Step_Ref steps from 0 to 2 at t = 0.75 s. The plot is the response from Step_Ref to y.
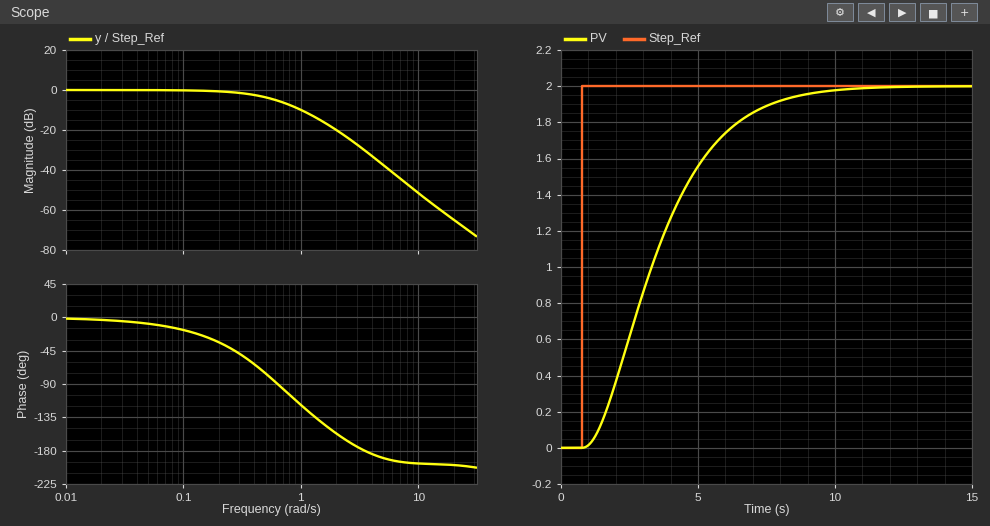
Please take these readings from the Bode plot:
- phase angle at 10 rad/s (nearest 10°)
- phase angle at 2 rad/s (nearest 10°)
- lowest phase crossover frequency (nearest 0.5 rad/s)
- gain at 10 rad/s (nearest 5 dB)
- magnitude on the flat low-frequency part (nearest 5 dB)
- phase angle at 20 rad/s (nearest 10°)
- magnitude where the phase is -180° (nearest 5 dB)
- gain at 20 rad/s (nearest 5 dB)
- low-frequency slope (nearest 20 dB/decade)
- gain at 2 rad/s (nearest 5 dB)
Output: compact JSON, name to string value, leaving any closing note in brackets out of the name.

{"phase angle at 10 rad/s": "-200°", "phase angle at 2 rad/s": "-160°", "lowest phase crossover frequency": "3.5 rad/s", "gain at 10 rad/s": "-50 dB", "magnitude on the flat low-frequency part": "0 dB", "phase angle at 20 rad/s": "-200°", "magnitude where the phase is -180°": "-30 dB", "gain at 20 rad/s": "-65 dB", "low-frequency slope": "0 dB/decade", "gain at 2 rad/s": "-20 dB"}
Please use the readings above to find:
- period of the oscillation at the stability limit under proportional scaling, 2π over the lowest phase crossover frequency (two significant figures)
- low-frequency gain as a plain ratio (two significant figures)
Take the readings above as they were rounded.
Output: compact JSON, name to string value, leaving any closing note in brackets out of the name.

{"period of the oscillation at the stability limit under proportional scaling, 2π over the lowest phase crossover frequency": "1.8 s", "low-frequency gain as a plain ratio": "1.0"}
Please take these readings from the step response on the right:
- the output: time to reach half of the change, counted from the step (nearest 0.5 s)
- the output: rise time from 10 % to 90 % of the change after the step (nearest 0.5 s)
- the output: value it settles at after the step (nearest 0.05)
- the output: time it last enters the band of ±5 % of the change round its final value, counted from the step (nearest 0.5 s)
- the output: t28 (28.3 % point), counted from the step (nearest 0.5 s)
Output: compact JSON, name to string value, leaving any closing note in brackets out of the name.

{"the output: time to reach half of the change, counted from the step": "2.5 s", "the output: rise time from 10 % to 90 % of the change after the step": "5.0 s", "the output: value it settles at after the step": "2.00", "the output: time it last enters the band of ±5 % of the change round its final value, counted from the step": "7.0 s", "the output: t28 (28.3 % point), counted from the step": "1.5 s"}
